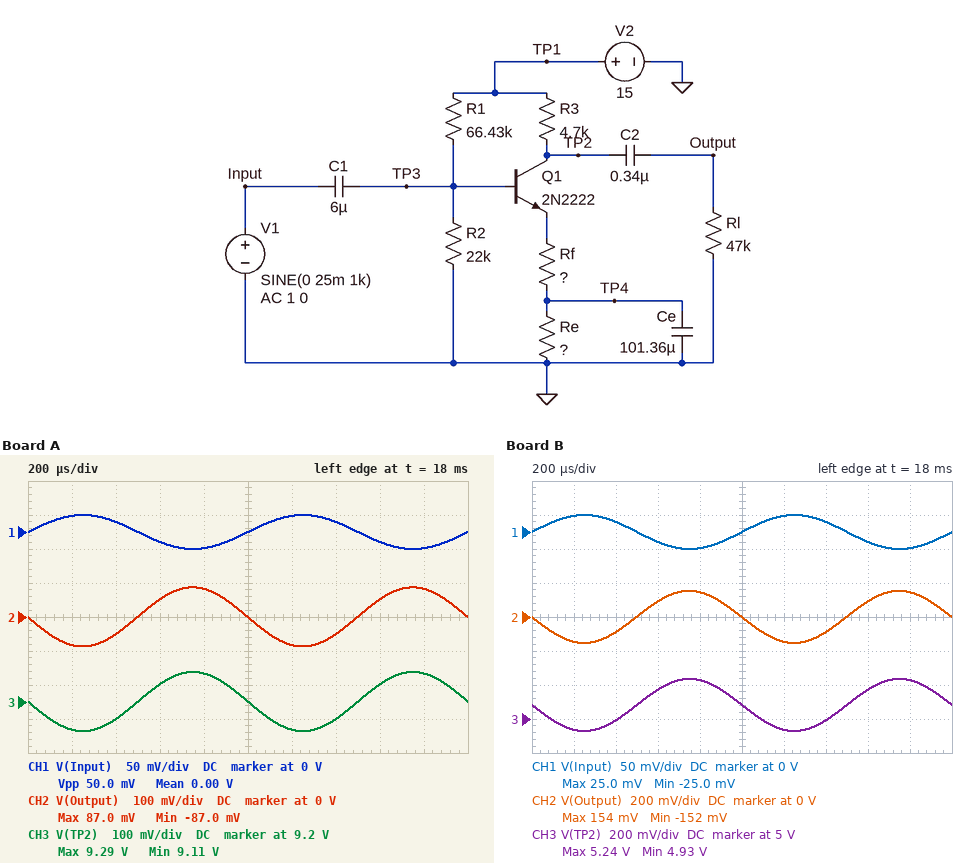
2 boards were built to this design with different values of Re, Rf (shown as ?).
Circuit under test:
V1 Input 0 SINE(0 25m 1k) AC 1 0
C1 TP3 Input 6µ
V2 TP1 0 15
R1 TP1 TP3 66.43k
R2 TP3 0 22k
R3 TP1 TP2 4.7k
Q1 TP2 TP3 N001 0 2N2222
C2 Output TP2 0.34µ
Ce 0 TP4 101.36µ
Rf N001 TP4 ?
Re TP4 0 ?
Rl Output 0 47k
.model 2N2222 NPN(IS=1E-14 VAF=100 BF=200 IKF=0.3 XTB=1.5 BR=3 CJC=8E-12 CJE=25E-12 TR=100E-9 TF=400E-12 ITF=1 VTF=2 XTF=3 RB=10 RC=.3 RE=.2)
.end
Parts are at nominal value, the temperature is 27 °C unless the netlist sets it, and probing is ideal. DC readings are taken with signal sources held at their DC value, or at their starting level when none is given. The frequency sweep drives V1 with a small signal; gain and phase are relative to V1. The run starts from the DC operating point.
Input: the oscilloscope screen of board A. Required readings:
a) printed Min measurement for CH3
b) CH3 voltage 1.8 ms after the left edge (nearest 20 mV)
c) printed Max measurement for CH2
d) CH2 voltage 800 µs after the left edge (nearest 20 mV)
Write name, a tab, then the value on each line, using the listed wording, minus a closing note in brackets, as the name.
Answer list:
printed Min measurement for CH3	9.11 V
CH3 voltage 1.8 ms after the left edge	9.28 V
printed Max measurement for CH2	87.0 mV
CH2 voltage 800 µs after the left edge	80 mV
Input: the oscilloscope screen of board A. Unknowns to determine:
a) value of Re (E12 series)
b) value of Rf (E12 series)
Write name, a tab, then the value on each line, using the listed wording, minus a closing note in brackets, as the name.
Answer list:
value of Re	1.2 kΩ
value of Rf	1.2 kΩ
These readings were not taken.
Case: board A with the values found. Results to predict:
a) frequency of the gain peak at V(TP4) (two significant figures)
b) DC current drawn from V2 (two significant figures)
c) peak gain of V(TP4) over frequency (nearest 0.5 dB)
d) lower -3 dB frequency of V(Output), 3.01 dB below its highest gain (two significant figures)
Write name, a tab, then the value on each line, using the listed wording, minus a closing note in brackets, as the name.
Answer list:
frequency of the gain peak at V(TP4)	2.1 Hz
DC current drawn from V2	1.4 mA
peak gain of V(TP4) over frequency	-10.5 dB
lower -3 dB frequency of V(Output), 3.01 dB below its highest gain	9.9 Hz
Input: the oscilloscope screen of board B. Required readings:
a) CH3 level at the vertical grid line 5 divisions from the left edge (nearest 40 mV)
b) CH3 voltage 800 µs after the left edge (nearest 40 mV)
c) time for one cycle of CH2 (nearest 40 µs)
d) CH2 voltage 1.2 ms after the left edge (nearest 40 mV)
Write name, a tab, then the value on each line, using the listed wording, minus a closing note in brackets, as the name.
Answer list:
CH3 level at the vertical grid line 5 divisions from the left edge	5.08 V
CH3 voltage 800 µs after the left edge	5.24 V
time for one cycle of CH2	1.00 ms
CH2 voltage 1.2 ms after the left edge	-160 mV
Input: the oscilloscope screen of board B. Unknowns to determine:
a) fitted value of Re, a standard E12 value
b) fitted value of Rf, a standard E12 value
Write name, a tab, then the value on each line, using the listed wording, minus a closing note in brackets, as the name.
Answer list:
fitted value of Re, a standard E12 value	680 Ω
fitted value of Rf, a standard E12 value	680 Ω
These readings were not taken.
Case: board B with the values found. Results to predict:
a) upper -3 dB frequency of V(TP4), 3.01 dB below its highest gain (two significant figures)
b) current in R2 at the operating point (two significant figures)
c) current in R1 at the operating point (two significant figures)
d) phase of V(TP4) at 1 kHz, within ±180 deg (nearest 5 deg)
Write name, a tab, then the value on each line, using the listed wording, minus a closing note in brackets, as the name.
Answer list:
upper -3 dB frequency of V(TP4), 3.01 dB below its highest gain	7.4 Hz
current in R2 at the operating point	160 µA
current in R1 at the operating point	170 µA
phase of V(TP4) at 1 kHz, within ±180 deg	-90 deg
